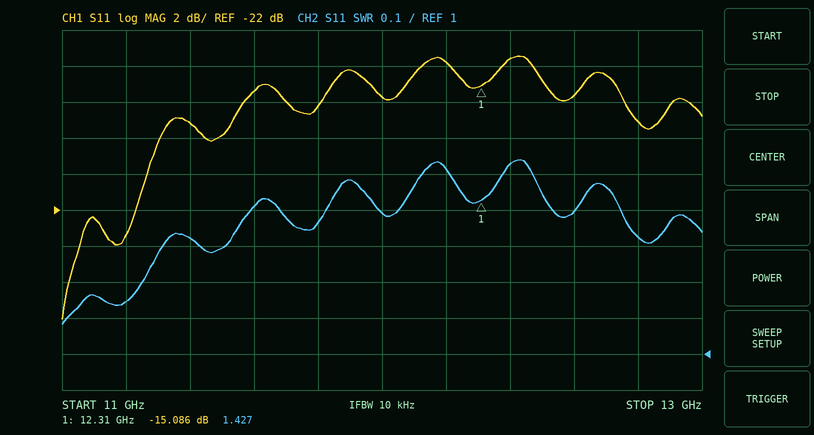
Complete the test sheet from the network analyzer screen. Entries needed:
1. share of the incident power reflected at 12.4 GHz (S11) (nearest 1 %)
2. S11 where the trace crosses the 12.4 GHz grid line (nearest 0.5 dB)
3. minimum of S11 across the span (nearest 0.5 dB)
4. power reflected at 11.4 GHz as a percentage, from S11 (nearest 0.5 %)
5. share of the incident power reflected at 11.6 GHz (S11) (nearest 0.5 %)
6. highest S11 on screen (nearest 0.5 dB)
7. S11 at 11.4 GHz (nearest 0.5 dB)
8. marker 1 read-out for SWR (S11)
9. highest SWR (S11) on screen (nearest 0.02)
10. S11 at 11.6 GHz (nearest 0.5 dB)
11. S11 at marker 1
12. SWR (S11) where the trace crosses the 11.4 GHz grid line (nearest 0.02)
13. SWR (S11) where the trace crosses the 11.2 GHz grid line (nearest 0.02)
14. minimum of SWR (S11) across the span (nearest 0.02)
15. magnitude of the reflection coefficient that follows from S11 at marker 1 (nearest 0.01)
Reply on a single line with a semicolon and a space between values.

4 %; -13.5 dB; -28.0 dB; 2.0 %; 3.0 %; -13.5 dB; -17.0 dB; 1.427; 1.54; -15.5 dB; -15.086 dB; 1.32; 1.14; 1.08; 0.18
